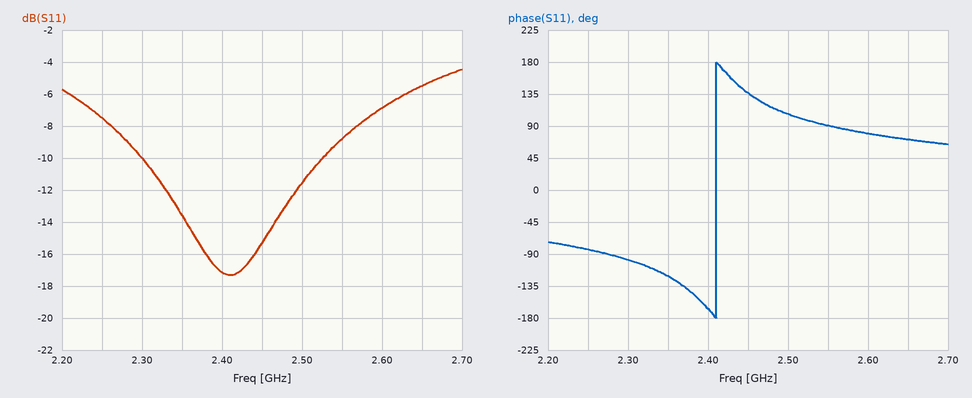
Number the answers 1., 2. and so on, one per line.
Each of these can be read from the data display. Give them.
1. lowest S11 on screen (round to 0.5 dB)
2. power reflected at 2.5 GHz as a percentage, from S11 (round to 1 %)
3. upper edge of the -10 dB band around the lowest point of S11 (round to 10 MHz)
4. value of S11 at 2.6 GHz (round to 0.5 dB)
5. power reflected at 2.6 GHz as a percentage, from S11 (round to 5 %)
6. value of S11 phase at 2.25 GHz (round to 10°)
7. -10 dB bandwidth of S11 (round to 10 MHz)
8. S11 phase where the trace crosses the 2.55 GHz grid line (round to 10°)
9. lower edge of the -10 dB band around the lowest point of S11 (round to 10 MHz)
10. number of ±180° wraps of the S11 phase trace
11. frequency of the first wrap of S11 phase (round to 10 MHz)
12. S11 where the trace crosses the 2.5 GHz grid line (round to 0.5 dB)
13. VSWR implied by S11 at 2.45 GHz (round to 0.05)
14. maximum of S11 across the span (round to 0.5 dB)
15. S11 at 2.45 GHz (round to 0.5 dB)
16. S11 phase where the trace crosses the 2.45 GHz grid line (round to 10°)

1. -17.5 dB
2. 7 %
3. 2.53 GHz
4. -7.0 dB
5. 20 %
6. -80°
7. 230 MHz
8. 90°
9. 2.30 GHz
10. 1
11. 2.41 GHz
12. -11.5 dB
13. 1.40
14. -4.5 dB
15. -15.5 dB
16. 140°
